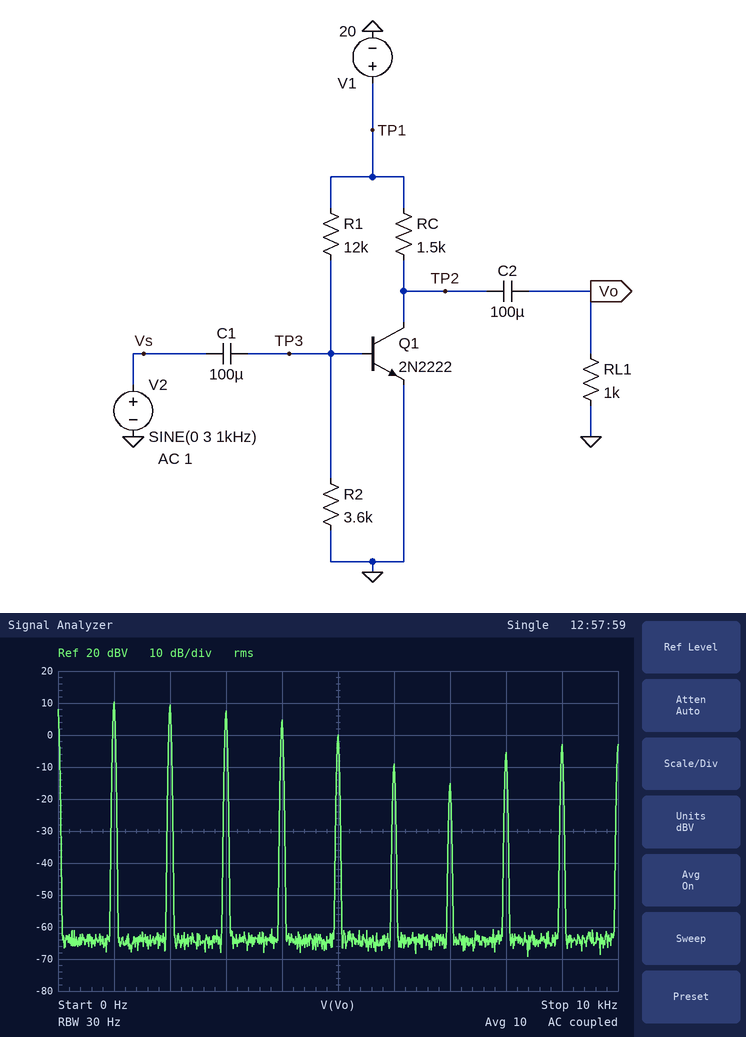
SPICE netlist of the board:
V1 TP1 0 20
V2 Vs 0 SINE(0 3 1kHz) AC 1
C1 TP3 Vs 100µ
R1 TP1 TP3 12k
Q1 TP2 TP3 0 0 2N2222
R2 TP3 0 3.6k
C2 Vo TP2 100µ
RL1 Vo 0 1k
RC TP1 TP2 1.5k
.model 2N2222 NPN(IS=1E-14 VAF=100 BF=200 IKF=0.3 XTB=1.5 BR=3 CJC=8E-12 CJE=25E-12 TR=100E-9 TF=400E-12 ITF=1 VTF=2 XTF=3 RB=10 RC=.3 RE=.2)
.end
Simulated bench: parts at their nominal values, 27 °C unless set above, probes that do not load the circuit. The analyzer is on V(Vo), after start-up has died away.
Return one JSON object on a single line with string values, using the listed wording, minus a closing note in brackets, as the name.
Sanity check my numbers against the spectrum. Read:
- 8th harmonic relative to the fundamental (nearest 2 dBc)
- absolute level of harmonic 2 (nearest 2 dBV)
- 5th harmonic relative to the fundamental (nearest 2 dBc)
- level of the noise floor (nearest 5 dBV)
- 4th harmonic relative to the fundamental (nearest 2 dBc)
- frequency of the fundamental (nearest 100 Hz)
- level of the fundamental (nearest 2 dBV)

{"8th harmonic relative to the fundamental": "-16 dBc", "absolute level of harmonic 2": "10 dBV", "5th harmonic relative to the fundamental": "-10 dBc", "level of the noise floor": "-65 dBV", "4th harmonic relative to the fundamental": "-6 dBc", "frequency of the fundamental": "1.0 kHz", "level of the fundamental": "10 dBV"}
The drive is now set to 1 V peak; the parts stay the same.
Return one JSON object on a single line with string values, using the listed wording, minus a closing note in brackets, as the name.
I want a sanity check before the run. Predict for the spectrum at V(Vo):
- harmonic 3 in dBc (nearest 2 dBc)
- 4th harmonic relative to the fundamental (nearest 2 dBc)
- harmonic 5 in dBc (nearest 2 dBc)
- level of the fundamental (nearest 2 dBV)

{"harmonic 3 in dBc": "-6 dBc", "4th harmonic relative to the fundamental": "-14 dBc", "harmonic 5 in dBc": "-32 dBc", "level of the fundamental": "12 dBV"}
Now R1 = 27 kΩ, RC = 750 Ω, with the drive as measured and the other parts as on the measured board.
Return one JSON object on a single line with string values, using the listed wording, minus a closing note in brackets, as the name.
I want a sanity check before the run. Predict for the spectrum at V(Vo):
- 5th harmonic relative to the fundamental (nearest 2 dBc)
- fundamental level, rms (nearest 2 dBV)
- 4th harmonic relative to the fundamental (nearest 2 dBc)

{"5th harmonic relative to the fundamental": "-6 dBc", "fundamental level, rms": "10 dBV", "4th harmonic relative to the fundamental": "-4 dBc"}
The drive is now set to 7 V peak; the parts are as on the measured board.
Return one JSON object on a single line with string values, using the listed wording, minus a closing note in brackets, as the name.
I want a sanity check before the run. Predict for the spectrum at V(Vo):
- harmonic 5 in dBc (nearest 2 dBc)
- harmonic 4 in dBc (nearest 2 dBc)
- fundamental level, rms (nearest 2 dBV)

{"harmonic 5 in dBc": "-6 dBc", "harmonic 4 in dBc": "-4 dBc", "fundamental level, rms": "10 dBV"}
